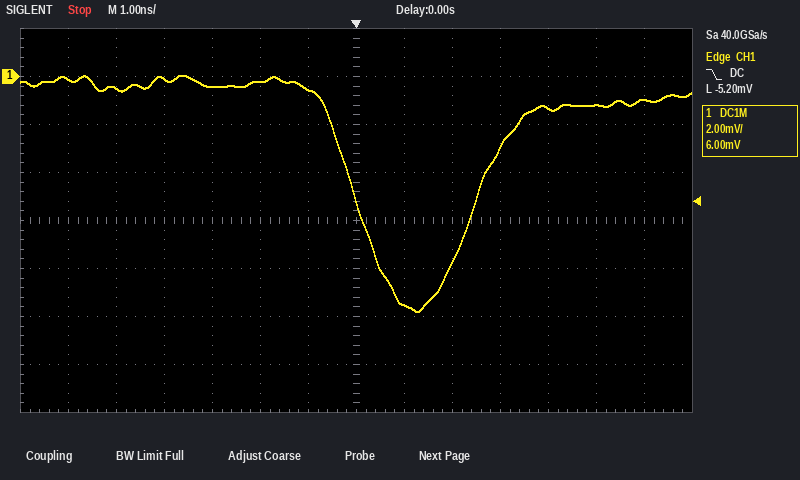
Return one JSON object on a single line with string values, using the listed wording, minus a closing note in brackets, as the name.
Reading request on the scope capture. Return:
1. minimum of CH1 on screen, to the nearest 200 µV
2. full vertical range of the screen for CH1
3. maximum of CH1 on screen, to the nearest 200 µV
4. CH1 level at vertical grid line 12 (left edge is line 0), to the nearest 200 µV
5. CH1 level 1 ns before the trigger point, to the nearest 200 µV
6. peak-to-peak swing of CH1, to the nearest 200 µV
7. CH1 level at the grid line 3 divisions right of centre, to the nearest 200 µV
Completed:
{"minimum of CH1 on screen, to the nearest 200 µV": "-9.8 mV", "full vertical range of the screen for CH1": "16 mV", "maximum of CH1 on screen, to the nearest 200 µV": "0.0 mV", "CH1 level at vertical grid line 12 (left edge is line 0), to the nearest 200 µV": "-1.2 mV", "CH1 level 1 ns before the trigger point, to the nearest 200 µV": "-600 µV", "peak-to-peak swing of CH1, to the nearest 200 µV": "9.8 mV", "CH1 level at the grid line 3 divisions right of centre, to the nearest 200 µV": "-3.0 mV"}
